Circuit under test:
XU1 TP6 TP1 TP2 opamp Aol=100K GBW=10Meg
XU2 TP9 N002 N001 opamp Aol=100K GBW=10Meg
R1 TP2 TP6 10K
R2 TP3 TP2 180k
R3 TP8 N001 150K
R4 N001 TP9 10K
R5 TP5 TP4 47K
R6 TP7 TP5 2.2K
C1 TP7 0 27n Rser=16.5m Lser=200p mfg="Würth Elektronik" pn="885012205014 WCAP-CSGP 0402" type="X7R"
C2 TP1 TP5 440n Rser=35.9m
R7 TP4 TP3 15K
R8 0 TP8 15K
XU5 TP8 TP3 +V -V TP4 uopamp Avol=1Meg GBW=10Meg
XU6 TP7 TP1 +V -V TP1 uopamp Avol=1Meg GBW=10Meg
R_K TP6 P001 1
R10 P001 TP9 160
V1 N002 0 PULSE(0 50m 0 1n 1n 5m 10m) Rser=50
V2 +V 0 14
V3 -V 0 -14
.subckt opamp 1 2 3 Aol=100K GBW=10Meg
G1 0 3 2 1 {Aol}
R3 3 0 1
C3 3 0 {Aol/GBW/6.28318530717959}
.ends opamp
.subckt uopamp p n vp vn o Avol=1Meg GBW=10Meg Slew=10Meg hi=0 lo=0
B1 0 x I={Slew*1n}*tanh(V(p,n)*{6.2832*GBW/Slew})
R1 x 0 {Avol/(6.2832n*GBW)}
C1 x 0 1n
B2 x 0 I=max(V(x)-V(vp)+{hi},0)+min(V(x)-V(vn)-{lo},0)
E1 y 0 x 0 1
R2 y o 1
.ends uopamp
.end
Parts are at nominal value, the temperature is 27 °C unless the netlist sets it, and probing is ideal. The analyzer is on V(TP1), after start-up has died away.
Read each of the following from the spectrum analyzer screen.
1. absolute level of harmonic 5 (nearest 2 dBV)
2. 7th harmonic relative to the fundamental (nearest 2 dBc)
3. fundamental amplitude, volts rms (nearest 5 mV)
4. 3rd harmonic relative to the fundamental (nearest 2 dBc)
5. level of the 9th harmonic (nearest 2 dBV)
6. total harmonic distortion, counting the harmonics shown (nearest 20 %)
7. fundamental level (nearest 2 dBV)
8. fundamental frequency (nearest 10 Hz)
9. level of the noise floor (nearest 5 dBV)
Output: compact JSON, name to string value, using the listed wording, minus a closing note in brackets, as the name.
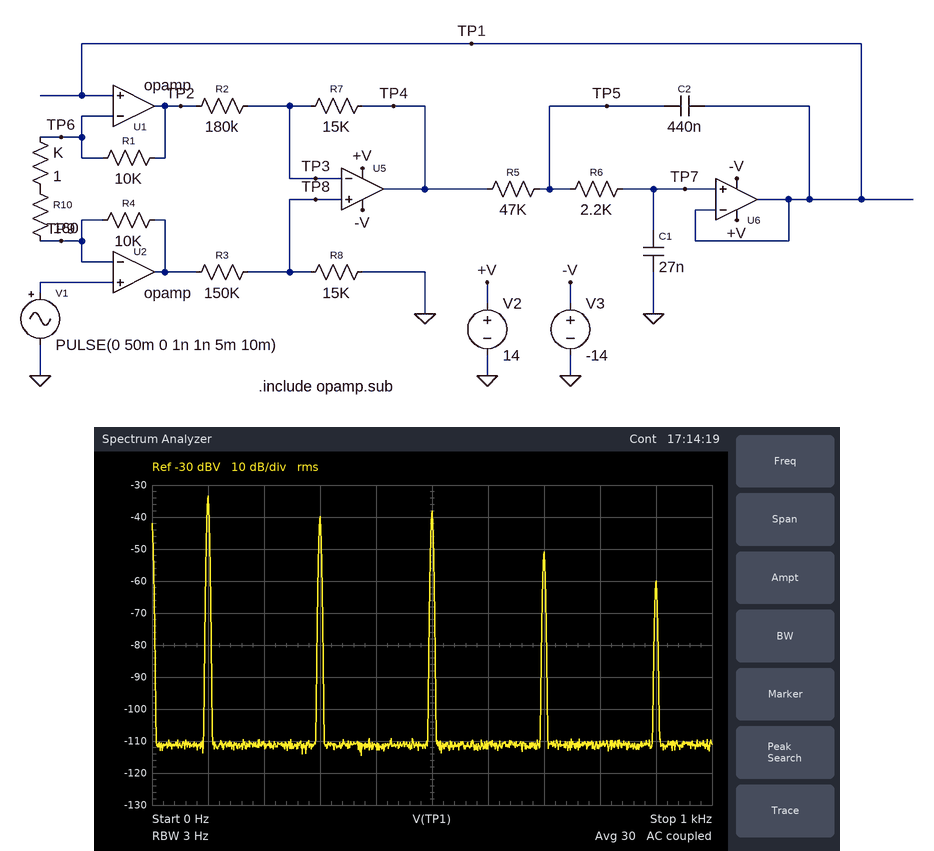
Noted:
{"absolute level of harmonic 5": "-38 dBV", "7th harmonic relative to the fundamental": "-18 dBc", "fundamental amplitude, volts rms": "20 mV", "3rd harmonic relative to the fundamental": "-6 dBc", "level of the 9th harmonic": "-60 dBV", "total harmonic distortion, counting the harmonics shown": "80 %", "fundamental level": "-34 dBV", "fundamental frequency": "100 Hz", "level of the noise floor": "-110 dBV"}
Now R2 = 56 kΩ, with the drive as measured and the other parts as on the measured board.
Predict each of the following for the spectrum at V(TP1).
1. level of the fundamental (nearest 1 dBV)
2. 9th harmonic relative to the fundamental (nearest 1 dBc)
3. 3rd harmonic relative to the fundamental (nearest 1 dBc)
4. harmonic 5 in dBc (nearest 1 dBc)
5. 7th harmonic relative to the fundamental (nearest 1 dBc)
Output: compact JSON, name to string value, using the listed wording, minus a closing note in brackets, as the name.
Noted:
{"level of the fundamental": "-33 dBV", "9th harmonic relative to the fundamental": "-15 dBc", "3rd harmonic relative to the fundamental": "-8 dBc", "harmonic 5 in dBc": "-9 dBc", "7th harmonic relative to the fundamental": "-4 dBc"}
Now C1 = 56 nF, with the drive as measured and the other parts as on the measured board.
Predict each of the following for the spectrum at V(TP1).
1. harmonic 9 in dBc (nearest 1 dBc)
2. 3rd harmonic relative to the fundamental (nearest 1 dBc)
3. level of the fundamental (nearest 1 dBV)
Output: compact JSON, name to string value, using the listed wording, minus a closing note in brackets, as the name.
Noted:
{"harmonic 9 in dBc": "-35 dBc", "3rd harmonic relative to the fundamental": "-4 dBc", "level of the fundamental": "-33 dBV"}
